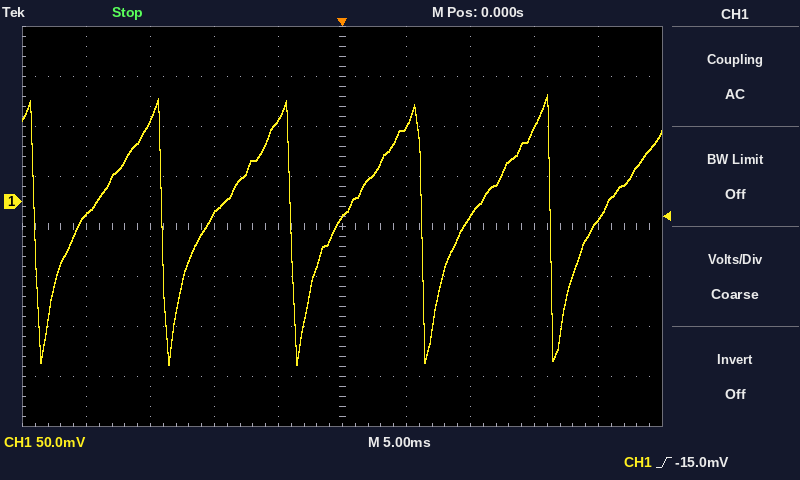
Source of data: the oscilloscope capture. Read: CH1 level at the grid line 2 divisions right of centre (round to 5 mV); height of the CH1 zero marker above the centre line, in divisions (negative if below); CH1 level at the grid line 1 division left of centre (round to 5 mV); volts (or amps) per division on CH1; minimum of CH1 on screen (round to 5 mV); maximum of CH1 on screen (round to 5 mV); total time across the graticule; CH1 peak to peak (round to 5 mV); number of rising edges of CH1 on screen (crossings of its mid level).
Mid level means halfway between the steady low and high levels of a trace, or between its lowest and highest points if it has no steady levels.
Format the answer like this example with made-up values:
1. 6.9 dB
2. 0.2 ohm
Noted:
1. -15 mV
2. +0.5 div
3. 80 mV
4. 50 mV
5. -165 mV
6. 105 mV
7. 50 ms
8. 270 mV
9. 5
